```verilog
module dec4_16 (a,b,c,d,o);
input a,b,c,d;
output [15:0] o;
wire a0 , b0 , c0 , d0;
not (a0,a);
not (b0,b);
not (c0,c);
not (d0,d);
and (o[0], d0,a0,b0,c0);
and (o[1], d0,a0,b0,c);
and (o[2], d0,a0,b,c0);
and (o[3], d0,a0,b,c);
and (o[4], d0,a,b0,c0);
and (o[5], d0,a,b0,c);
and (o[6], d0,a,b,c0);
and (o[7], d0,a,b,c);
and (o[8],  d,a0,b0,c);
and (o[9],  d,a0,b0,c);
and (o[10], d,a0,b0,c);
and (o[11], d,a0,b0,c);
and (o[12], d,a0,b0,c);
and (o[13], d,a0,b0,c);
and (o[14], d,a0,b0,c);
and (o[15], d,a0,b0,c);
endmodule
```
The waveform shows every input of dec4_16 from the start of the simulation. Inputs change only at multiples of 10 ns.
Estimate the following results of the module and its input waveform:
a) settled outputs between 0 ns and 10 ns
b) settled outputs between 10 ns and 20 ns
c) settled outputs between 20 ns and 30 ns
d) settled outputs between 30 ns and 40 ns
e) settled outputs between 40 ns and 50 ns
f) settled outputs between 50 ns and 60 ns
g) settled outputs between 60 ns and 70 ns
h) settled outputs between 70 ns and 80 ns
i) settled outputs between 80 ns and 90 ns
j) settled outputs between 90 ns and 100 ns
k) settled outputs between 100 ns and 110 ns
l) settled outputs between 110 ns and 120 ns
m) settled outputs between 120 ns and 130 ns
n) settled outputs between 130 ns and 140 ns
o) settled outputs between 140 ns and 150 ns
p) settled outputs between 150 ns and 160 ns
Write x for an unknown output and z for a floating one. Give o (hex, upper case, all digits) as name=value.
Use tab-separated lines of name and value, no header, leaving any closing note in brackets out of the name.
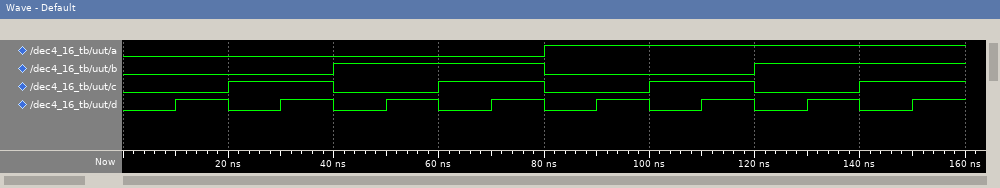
settled outputs between 0 ns and 10 ns	o=0001
settled outputs between 10 ns and 20 ns	o=0000
settled outputs between 20 ns and 30 ns	o=0002
settled outputs between 30 ns and 40 ns	o=FF00
settled outputs between 40 ns and 50 ns	o=0004
settled outputs between 50 ns and 60 ns	o=0000
settled outputs between 60 ns and 70 ns	o=0008
settled outputs between 70 ns and 80 ns	o=0000
settled outputs between 80 ns and 90 ns	o=0010
settled outputs between 90 ns and 100 ns	o=0000
settled outputs between 100 ns and 110 ns	o=0020
settled outputs between 110 ns and 120 ns	o=0000
settled outputs between 120 ns and 130 ns	o=0040
settled outputs between 130 ns and 140 ns	o=0000
settled outputs between 140 ns and 150 ns	o=0080
settled outputs between 150 ns and 160 ns	o=0000
